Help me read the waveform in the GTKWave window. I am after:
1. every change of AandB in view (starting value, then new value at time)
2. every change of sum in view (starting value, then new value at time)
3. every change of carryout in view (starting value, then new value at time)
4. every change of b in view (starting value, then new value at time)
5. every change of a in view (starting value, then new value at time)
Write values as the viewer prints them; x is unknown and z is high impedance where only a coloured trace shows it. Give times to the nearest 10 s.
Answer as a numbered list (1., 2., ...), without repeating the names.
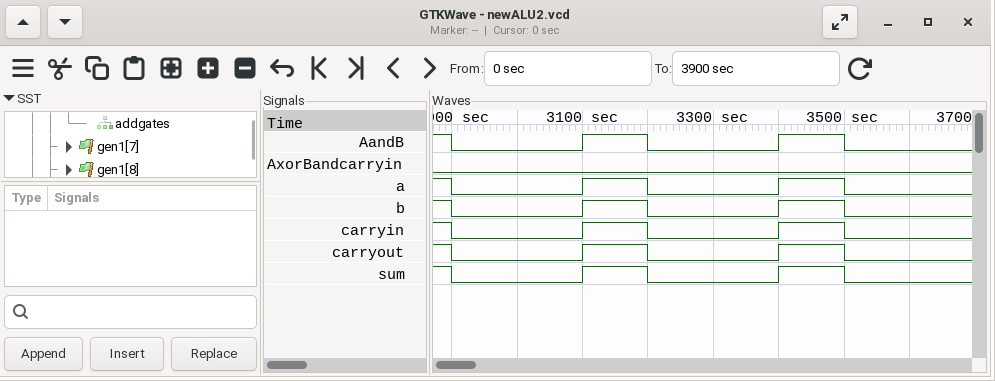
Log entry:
1. 1, 0 at 2900 s, 1 at 3100 s, 0 at 3200 s, 1 at 3400 s, 0 at 3500 s
2. 1, 0 at 2900 s, 1 at 3100 s, 0 at 3200 s, 1 at 3400 s, 0 at 3500 s
3. 1, 0 at 2900 s, 1 at 3100 s, 0 at 3200 s, 1 at 3400 s, 0 at 3500 s
4. 1, 0 at 2900 s, 1 at 3100 s, 0 at 3200 s, 1 at 3400 s, 0 at 3500 s
5. 1, 0 at 2900 s, 1 at 3100 s, 0 at 3200 s, 1 at 3400 s, 0 at 3500 s
